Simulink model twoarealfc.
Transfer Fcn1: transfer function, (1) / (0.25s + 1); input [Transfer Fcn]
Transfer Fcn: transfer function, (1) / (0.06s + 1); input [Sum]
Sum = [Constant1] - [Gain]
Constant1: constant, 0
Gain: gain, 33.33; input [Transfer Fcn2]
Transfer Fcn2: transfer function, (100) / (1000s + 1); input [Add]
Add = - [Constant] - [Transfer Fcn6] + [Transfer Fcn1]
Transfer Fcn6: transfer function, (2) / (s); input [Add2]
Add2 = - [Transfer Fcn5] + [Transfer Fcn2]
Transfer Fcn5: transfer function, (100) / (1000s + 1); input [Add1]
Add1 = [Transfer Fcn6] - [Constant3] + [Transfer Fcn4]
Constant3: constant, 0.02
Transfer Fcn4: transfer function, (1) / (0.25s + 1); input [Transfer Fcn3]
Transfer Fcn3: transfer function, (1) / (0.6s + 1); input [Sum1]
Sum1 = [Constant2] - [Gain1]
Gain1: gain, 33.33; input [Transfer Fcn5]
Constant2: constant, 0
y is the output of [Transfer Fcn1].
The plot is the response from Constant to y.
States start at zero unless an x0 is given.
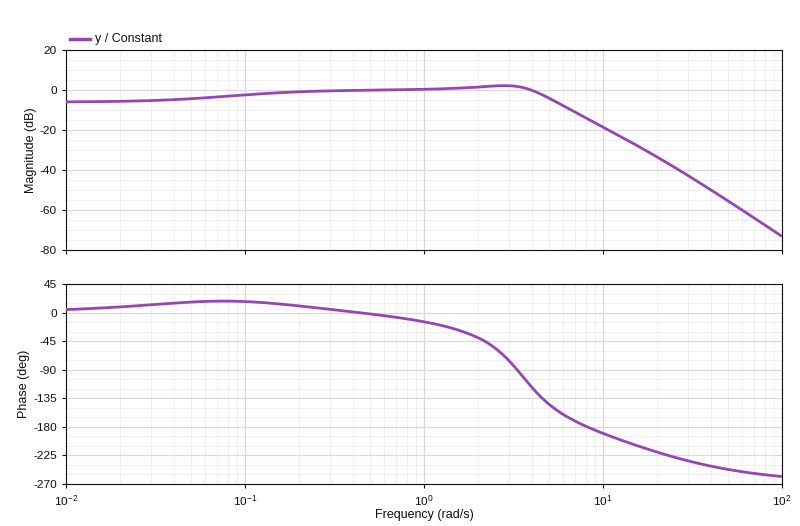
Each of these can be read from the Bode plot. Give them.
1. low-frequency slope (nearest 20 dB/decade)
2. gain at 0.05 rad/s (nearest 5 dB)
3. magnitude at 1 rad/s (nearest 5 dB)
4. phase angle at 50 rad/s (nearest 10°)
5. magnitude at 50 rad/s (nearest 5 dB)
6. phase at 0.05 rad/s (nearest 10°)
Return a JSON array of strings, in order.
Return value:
["0 dB/decade", "-5 dB", "0 dB", "-250°", "-55 dB", "20°"]
